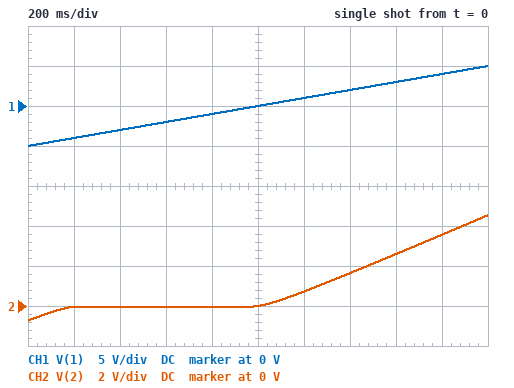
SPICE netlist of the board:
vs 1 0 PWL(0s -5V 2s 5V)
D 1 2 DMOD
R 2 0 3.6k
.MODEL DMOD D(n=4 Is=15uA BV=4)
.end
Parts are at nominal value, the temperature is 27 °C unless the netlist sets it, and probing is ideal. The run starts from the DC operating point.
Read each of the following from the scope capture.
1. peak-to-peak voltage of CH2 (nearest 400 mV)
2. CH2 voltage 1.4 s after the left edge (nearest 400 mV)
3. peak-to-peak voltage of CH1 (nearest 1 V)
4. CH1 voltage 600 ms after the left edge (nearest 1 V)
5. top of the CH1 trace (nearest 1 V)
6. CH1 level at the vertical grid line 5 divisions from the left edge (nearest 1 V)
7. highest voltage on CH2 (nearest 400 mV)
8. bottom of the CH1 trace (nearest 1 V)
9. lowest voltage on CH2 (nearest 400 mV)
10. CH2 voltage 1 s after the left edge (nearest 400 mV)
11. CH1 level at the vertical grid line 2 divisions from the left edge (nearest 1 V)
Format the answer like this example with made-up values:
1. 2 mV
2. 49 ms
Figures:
1. 5.2 V
2. 1.6 V
3. 10 V
4. -2 V
5. 5 V
6. 0 V
7. 4.4 V
8. -5 V
9. -800 mV
10. 0 V
11. -3 V
